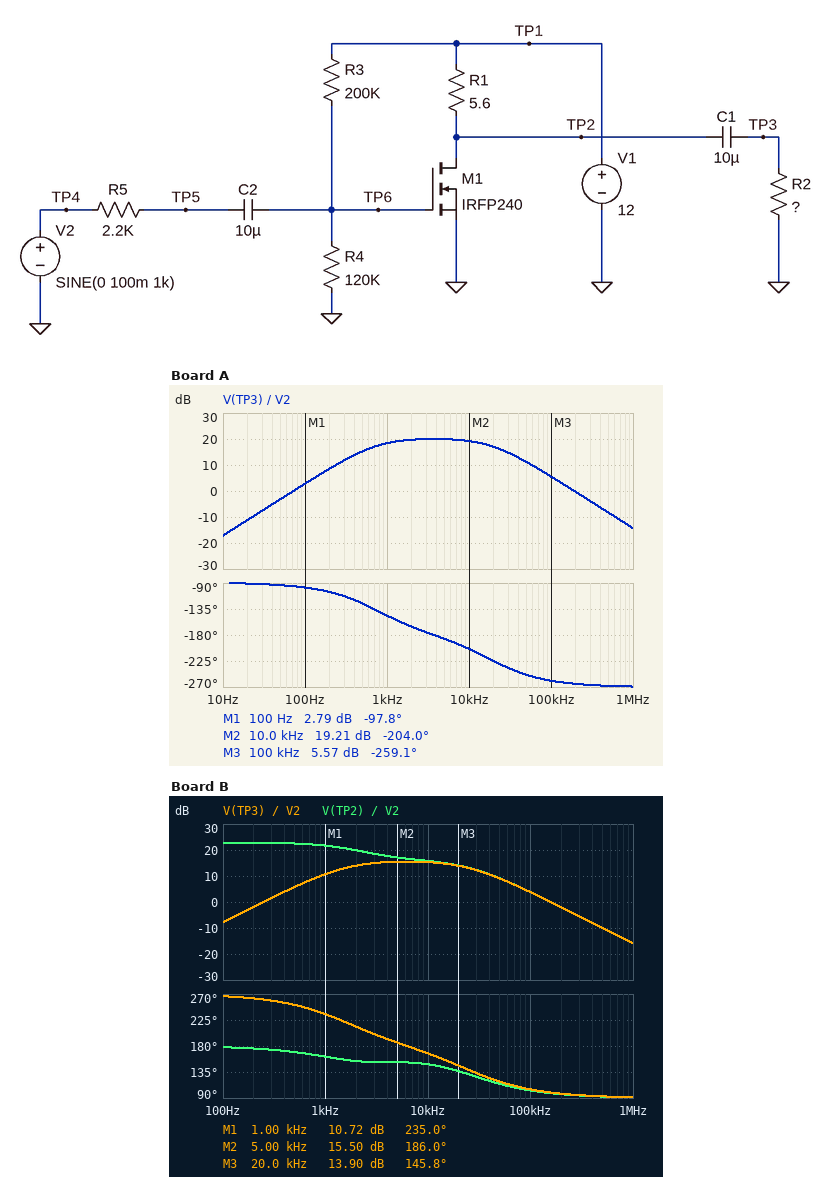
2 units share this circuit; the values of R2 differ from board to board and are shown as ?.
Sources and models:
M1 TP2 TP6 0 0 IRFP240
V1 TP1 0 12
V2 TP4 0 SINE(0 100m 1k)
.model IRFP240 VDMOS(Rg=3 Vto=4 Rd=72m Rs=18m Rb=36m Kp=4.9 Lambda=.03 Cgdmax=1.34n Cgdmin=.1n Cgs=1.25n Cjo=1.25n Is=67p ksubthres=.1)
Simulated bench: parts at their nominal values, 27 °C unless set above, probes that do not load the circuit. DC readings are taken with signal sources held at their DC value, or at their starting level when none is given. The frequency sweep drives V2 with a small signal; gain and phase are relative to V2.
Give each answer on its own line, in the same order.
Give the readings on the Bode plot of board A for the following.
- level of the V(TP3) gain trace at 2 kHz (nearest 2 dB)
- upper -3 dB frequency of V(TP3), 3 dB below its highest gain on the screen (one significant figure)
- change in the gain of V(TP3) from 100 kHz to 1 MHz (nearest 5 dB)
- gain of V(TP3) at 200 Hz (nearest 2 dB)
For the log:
20 dB
20 kHz
-20 dB
8 dB
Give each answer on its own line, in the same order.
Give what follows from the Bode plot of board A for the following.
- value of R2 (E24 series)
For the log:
16 Ω
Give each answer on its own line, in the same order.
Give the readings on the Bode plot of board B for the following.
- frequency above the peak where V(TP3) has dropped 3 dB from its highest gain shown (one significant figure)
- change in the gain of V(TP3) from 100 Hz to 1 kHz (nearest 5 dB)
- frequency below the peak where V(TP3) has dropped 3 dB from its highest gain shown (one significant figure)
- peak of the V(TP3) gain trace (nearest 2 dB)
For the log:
30 kHz
20 dB
1 kHz
16 dB
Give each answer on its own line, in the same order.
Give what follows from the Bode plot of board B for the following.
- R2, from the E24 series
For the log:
4.7 Ω
